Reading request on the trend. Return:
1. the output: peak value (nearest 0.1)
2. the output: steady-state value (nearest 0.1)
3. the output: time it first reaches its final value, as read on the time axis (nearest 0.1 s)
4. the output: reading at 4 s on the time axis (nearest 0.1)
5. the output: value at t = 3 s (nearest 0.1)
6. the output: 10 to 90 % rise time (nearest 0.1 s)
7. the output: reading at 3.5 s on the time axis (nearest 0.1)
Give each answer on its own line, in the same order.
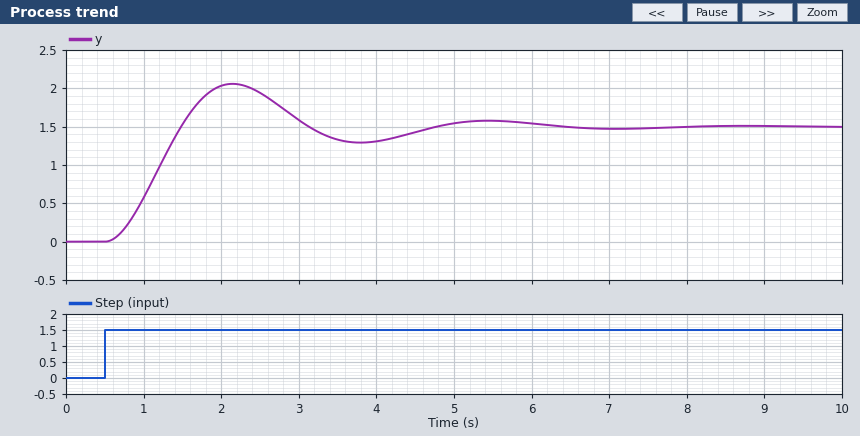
2.1
1.5
1.5 s
1.3
1.6
0.7 s
1.3
